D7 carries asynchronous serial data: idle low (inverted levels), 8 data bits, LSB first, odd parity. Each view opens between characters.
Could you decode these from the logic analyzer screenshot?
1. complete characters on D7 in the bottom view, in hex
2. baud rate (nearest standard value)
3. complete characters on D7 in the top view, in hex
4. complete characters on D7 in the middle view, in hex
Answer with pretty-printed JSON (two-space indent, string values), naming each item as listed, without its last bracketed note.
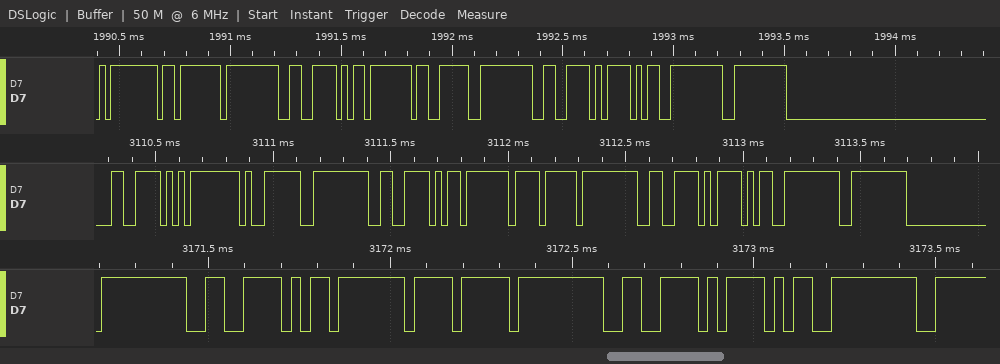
{
  "complete characters on D7 in the bottom view, in hex": "00, 86, 02, 08, 00, 86, 28, 00",
  "baud rate": "38400 baud",
  "complete characters on D7 in the top view, in hex": "01, 02, 00, 86, 02, 06, 00, 86, 28, 00, 00",
  "complete characters on D7 in the middle view, in hex": "86, 01, 03, 00, 86, 02, 08, 00, 86, 28, 00, 00"
}
